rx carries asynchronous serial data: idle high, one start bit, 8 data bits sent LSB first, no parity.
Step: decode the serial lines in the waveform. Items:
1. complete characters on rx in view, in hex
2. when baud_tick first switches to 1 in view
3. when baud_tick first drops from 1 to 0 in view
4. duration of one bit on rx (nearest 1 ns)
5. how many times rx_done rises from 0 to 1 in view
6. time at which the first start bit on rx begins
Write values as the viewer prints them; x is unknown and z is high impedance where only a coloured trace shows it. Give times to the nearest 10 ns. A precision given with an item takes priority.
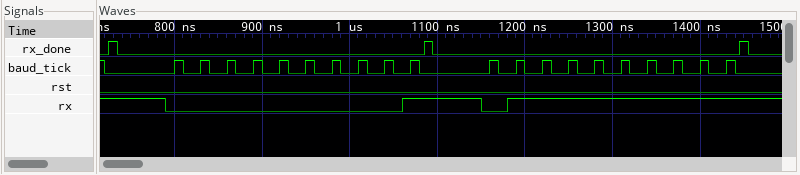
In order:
00, FF
800 ns
720 ns
30 ns
3
790 ns
